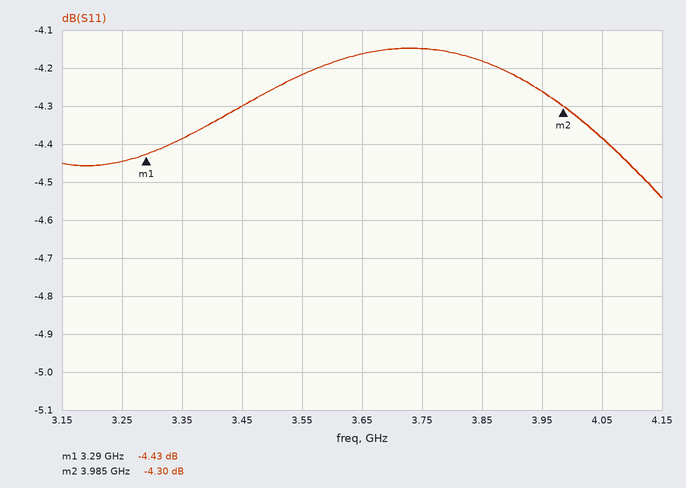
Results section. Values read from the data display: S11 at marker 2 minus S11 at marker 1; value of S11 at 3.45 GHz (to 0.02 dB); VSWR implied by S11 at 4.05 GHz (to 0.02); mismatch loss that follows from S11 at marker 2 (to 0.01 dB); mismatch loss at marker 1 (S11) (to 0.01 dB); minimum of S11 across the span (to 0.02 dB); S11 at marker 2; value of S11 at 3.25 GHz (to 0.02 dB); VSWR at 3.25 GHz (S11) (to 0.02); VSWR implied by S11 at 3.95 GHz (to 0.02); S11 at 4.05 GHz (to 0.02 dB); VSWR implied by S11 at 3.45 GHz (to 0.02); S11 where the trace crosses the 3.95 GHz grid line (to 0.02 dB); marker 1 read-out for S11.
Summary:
0.13 dB
-4.30 dB
4.04
2.02 dB
1.94 dB
-4.54 dB
-4.30 dB
-4.44 dB
4.00
4.16
-4.38 dB
4.12
-4.26 dB
-4.43 dB
